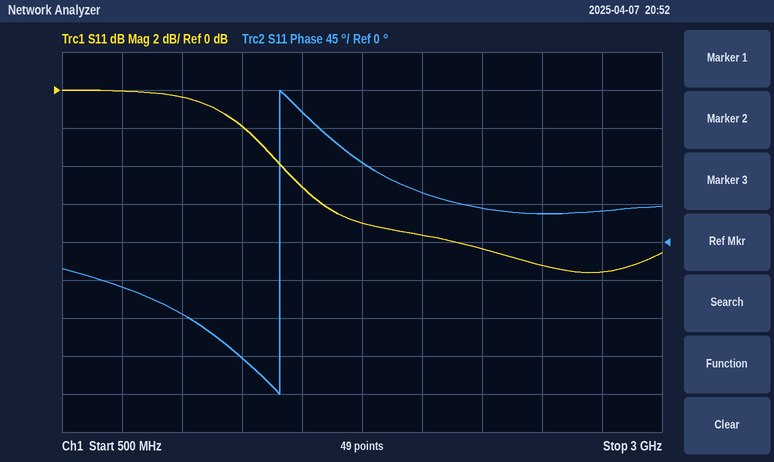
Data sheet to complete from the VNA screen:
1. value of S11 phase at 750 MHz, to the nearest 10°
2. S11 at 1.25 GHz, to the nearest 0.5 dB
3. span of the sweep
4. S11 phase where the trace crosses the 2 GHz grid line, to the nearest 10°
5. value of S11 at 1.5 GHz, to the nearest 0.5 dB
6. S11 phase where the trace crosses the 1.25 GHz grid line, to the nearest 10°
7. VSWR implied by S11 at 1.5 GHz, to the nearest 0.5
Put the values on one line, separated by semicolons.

-50°; -2.0 dB; 2.5 GHz; 60°; -5.0 dB; -140°; 3.5
